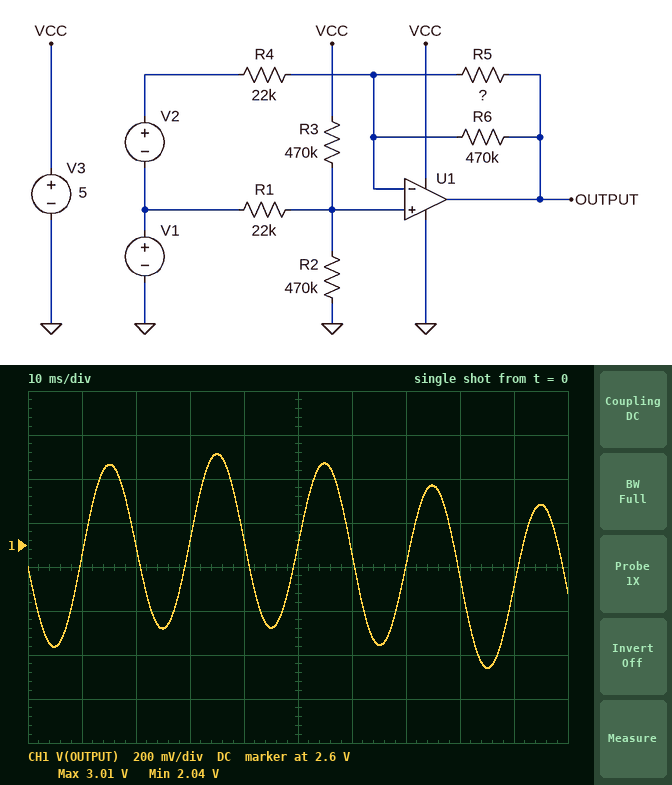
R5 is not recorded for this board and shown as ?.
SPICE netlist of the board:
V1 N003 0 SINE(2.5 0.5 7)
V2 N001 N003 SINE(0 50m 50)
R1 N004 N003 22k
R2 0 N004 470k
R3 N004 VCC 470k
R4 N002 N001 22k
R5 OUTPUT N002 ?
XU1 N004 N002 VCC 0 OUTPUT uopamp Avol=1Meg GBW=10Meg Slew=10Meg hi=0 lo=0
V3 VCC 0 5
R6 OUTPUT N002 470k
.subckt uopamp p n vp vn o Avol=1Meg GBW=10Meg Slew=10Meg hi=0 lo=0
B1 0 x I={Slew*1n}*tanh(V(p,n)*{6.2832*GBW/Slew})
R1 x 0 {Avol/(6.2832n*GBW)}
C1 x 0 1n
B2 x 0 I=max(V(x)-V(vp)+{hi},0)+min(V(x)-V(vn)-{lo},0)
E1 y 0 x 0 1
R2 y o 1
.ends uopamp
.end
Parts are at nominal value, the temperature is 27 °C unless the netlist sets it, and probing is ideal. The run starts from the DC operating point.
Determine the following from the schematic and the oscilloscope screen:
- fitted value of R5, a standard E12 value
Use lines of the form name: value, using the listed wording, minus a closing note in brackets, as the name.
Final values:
fitted value of R5, a standard E12 value: 270 kΩ
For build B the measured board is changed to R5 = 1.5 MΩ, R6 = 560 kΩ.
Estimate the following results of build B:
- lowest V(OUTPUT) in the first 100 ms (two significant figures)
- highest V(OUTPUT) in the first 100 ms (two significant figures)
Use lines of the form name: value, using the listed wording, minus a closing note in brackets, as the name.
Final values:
lowest V(OUTPUT) in the first 100 ms: 1.3 V
highest V(OUTPUT) in the first 100 ms: 3.7 V
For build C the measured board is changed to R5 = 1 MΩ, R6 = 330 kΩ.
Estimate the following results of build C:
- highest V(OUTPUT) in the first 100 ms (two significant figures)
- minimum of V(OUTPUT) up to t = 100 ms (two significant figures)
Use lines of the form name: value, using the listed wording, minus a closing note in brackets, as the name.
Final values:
highest V(OUTPUT) in the first 100 ms: 3.1 V
minimum of V(OUTPUT) up to t = 100 ms: 1.9 V
